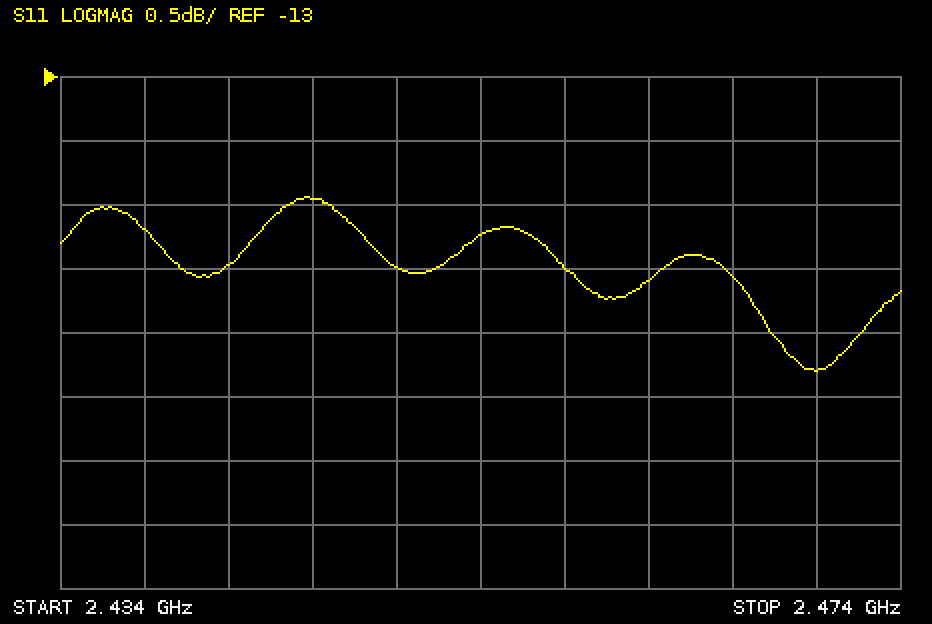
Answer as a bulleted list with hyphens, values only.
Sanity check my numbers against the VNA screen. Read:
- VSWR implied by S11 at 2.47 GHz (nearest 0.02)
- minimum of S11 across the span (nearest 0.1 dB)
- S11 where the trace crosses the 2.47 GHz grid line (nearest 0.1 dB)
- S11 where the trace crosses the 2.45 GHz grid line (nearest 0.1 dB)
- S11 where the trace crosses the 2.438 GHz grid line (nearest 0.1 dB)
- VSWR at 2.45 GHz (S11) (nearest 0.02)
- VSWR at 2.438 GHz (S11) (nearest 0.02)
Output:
- 1.42
- -15.3 dB
- -15.3 dB
- -14.5 dB
- -14.2 dB
- 1.46
- 1.48
